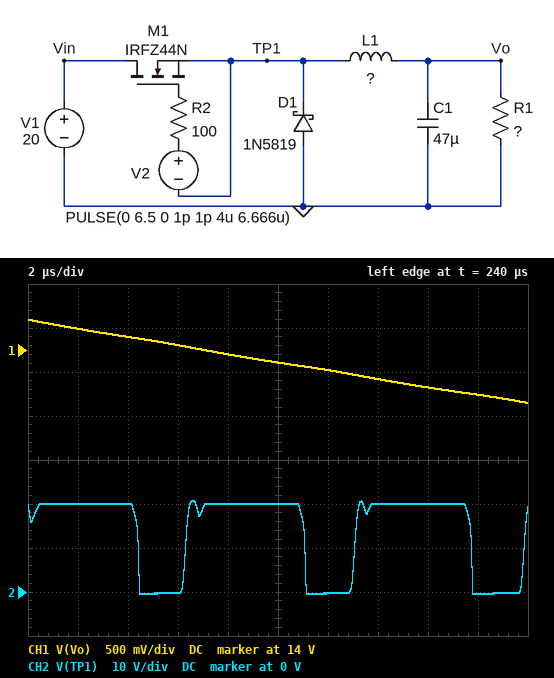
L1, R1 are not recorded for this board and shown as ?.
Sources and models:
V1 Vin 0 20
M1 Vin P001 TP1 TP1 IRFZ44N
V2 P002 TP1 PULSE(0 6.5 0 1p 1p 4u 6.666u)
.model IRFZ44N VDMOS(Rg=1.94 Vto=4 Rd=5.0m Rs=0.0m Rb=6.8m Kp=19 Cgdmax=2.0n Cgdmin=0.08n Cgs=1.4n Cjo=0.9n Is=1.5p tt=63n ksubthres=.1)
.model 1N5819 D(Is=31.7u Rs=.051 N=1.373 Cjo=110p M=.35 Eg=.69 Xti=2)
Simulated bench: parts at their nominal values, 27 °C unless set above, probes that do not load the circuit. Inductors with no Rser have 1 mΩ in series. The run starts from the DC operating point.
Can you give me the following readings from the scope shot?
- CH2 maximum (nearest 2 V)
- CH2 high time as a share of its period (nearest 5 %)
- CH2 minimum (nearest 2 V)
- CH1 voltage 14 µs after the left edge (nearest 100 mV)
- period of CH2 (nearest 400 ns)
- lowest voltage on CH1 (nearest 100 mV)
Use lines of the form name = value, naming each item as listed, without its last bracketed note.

CH2 maximum = 20 V
CH2 high time as a share of its period = 70 %
CH2 minimum = 0 V
CH1 voltage 14 µs after the left edge = 13.7 V
period of CH2 = 6.8 µs
lowest voltage on CH1 = 13.4 V
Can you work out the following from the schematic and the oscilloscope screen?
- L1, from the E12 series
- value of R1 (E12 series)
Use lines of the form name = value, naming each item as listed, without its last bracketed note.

L1, from the E12 series = 47 µH
value of R1 = 5.6 Ω
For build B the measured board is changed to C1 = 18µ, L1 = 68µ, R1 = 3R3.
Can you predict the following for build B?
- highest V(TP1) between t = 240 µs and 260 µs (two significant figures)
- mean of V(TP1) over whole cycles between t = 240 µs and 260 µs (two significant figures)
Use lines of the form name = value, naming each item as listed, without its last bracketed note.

highest V(TP1) between t = 240 µs and 260 µs = 20 V
mean of V(TP1) over whole cycles between t = 240 µs and 260 µs = 12 V
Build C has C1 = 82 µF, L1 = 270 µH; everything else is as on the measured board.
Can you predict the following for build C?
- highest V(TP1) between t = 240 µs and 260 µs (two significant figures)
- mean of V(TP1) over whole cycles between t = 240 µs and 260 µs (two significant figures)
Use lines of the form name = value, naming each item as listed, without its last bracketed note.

highest V(TP1) between t = 240 µs and 260 µs = 20 V
mean of V(TP1) over whole cycles between t = 240 µs and 260 µs = 11 V
